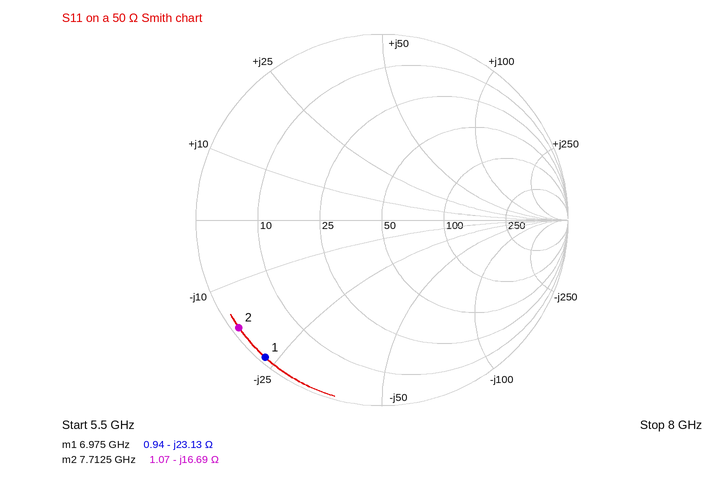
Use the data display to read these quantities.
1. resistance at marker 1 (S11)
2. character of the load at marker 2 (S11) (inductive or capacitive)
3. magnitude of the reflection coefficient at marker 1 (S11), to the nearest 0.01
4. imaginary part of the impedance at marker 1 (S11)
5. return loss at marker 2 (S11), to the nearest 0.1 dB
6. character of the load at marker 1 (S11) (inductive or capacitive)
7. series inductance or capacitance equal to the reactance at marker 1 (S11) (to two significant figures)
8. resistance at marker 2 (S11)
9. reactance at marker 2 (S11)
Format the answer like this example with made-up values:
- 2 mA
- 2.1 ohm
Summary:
- 0.94 Ω
- capacitive
- 0.97
- -23.13 Ω
- 0.3 dB
- capacitive
- 990 fF
- 1.07 Ω
- -16.69 Ω
